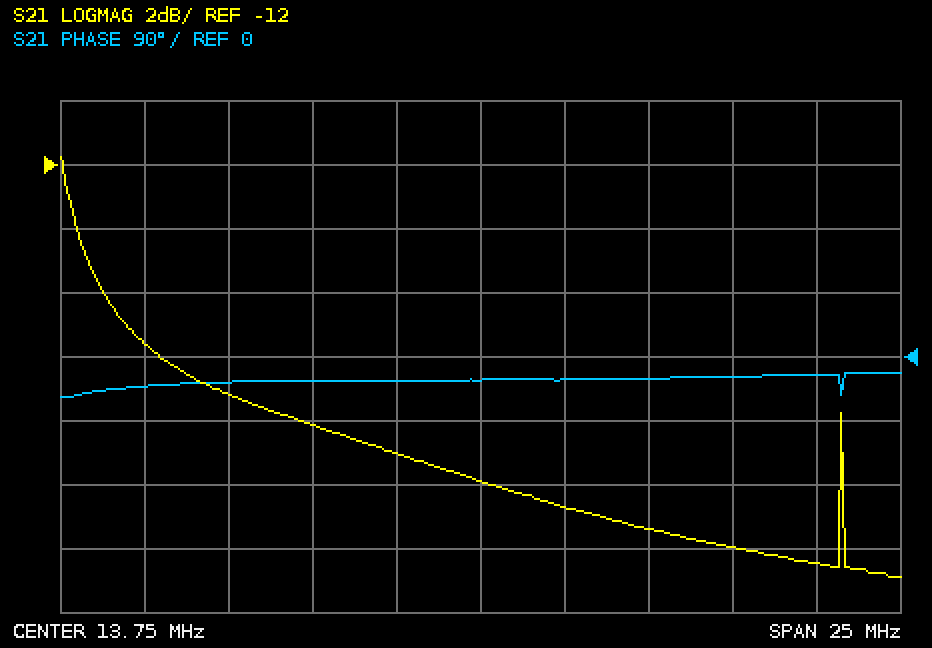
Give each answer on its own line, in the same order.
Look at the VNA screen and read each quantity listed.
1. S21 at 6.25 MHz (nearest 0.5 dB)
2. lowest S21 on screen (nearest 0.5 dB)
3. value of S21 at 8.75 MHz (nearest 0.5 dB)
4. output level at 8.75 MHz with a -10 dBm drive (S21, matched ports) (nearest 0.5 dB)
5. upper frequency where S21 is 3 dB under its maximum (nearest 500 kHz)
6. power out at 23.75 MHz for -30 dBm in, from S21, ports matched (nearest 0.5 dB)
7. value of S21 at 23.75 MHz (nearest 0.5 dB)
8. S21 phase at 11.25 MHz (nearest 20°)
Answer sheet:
-19.0 dB
-25.0 dB
-20.0 dB
-30.0 dBm
2.0 MHz
-54.5 dBm
-24.5 dB
-40°
